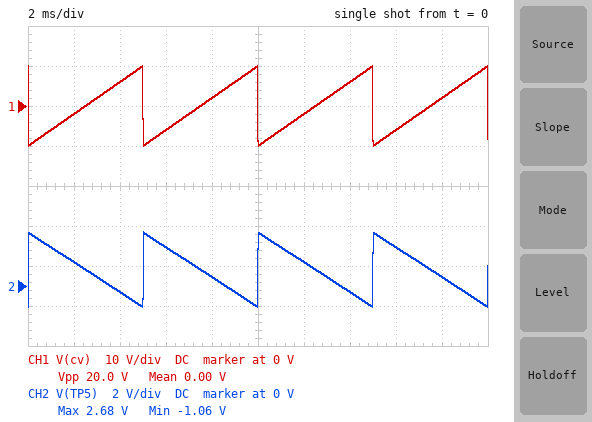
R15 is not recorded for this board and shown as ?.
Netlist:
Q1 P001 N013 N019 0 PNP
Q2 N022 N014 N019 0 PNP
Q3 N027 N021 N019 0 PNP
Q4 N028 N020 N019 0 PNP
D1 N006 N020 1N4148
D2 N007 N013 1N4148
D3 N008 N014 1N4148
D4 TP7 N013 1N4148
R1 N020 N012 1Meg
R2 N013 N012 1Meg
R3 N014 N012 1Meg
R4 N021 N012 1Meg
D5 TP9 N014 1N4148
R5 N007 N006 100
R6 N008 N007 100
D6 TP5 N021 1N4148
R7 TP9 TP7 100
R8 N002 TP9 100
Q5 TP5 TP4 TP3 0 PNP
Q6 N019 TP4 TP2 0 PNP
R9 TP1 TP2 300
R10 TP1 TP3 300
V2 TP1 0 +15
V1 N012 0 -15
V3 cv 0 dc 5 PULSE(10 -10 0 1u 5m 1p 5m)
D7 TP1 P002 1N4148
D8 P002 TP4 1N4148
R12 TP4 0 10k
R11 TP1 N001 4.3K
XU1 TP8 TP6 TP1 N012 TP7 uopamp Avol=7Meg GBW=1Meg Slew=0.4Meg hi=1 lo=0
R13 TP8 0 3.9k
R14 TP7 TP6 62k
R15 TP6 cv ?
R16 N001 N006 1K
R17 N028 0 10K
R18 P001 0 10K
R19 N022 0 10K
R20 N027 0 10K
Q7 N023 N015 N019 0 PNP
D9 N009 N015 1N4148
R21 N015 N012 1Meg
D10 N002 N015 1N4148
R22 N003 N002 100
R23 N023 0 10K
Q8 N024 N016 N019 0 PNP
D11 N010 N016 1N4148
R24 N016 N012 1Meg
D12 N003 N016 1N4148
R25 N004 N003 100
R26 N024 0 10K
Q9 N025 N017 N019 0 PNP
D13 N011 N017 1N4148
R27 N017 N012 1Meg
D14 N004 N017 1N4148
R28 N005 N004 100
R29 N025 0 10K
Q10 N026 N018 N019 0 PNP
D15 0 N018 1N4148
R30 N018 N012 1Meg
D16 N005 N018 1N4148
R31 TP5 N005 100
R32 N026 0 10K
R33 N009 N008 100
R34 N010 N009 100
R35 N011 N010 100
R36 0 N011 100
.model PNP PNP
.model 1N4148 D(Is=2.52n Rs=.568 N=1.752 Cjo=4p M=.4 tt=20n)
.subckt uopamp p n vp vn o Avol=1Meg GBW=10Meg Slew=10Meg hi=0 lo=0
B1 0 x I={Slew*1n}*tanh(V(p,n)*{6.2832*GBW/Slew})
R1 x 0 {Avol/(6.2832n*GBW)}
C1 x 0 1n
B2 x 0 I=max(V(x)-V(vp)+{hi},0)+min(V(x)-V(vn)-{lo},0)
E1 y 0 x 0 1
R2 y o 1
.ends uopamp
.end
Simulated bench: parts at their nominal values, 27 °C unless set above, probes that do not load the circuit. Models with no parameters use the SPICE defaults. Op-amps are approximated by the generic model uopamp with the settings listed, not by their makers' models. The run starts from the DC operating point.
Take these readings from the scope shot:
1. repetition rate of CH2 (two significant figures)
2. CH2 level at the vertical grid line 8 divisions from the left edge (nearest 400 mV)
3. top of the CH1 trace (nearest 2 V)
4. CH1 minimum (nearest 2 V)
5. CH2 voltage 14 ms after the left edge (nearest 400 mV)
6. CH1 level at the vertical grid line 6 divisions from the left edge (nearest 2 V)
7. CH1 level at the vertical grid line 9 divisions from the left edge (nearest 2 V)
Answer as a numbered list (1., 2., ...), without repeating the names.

1. 200 Hz
2. 2.0 V
3. 10 V
4. -10 V
5. -400 mV
6. -2 V
7. 2 V
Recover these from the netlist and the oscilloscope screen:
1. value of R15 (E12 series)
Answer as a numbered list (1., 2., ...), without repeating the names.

1. 330 kΩ
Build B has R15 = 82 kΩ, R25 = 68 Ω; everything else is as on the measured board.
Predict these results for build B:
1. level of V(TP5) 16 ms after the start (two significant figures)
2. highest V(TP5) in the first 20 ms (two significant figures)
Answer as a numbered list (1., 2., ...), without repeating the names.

1. 5.3 V
2. 8.2 V
